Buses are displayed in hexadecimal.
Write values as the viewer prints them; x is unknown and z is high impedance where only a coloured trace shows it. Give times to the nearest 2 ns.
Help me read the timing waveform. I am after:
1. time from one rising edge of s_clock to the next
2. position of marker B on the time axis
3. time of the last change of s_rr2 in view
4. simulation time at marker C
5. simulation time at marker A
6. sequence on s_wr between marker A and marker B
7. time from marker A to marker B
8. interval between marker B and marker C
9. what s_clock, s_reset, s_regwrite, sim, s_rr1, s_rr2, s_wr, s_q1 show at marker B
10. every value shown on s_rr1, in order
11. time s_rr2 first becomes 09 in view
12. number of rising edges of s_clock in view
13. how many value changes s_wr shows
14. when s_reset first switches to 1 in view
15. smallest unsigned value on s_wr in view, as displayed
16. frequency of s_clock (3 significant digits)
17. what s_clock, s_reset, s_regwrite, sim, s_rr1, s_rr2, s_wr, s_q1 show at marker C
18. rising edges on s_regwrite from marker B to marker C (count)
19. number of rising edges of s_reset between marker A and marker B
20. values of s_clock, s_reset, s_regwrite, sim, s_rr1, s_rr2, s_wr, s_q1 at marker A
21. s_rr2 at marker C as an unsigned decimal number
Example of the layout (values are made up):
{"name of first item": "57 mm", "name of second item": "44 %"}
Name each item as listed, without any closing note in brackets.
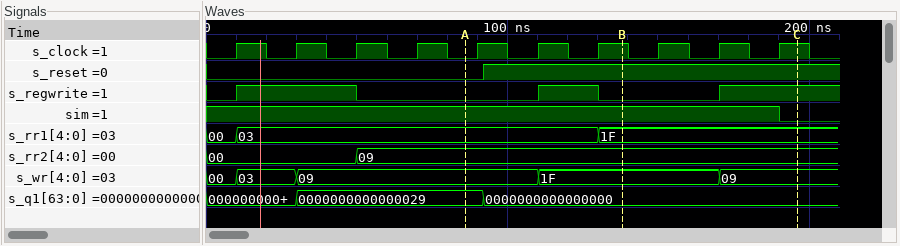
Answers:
{"time from one rising edge of s_clock to the next": "20 ns", "position of marker B on the time axis": "138 ns", "time of the last change of s_rr2 in view": "50 ns", "simulation time at marker C": "196 ns", "simulation time at marker A": "86 ns", "sequence on s_wr between marker A and marker B": "09, 1F", "time from marker A to marker B": "52 ns", "interval between marker B and marker C": "58 ns", "what s_clock, s_reset, s_regwrite, sim, s_rr1, s_rr2, s_wr, s_q1 show at marker B": "s_clock=1, s_reset=1, s_regwrite=0, sim=1, s_rr1=1F, s_rr2=09, s_wr=1F, s_q1=0000000000000000", "every value shown on s_rr1, in order": "00, 03, 1F", "time s_rr2 first becomes 09 in view": "50 ns", "number of rising edges of s_clock in view": "10", "how many value changes s_wr shows": "4", "when s_reset first switches to 1 in view": "92 ns", "smallest unsigned value on s_wr in view, as displayed": "00", "frequency of s_clock": "50.0 MHz", "what s_clock, s_reset, s_regwrite, sim, s_rr1, s_rr2, s_wr, s_q1 show at marker C": "s_clock=1, s_reset=1, s_regwrite=1, sim=0, s_rr1=1F, s_rr2=09, s_wr=09, s_q1=0000000000000000", "rising edges on s_regwrite from marker B to marker C": "1", "number of rising edges of s_reset between marker A and marker B": "1", "values of s_clock, s_reset, s_regwrite, sim, s_rr1, s_rr2, s_wr, s_q1 at marker A": "s_clock=0, s_reset=0, s_regwrite=0, sim=1, s_rr1=03, s_rr2=09, s_wr=09, s_q1=0000000000000029", "s_rr2 at marker C as an unsigned decimal number": "9"}
